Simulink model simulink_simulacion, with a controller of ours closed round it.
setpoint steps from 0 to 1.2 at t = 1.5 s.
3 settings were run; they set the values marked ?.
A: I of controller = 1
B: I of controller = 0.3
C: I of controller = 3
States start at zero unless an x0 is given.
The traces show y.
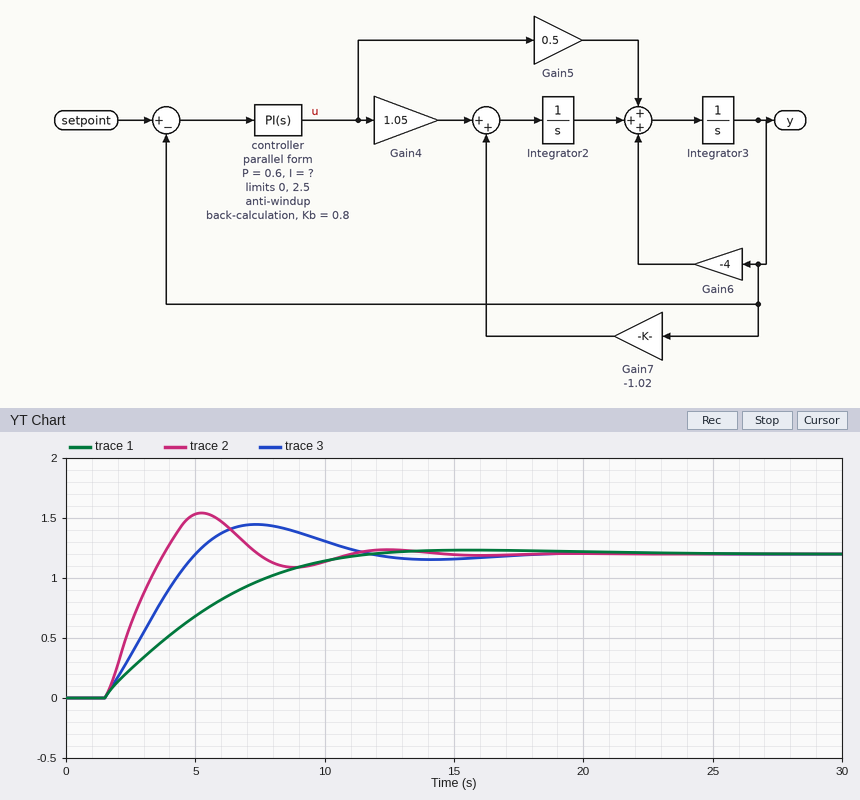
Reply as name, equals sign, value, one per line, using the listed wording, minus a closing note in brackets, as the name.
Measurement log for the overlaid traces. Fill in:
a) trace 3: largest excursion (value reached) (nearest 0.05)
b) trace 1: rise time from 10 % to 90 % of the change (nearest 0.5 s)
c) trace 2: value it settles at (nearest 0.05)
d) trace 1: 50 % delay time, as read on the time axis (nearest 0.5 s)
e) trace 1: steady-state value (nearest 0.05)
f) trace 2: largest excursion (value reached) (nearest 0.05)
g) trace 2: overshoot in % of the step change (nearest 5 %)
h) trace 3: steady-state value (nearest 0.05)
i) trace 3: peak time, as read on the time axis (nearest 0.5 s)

trace 3: largest excursion (value reached) = 1.45
trace 1: rise time from 10 % to 90 % of the change = 7.0 s
trace 2: value it settles at = 1.20
trace 1: 50 % delay time, as read on the time axis = 4.5 s
trace 1: steady-state value = 1.20
trace 2: largest excursion (value reached) = 1.55
trace 2: overshoot in % of the step change = 30 %
trace 3: steady-state value = 1.20
trace 3: peak time, as read on the time axis = 7.5 s
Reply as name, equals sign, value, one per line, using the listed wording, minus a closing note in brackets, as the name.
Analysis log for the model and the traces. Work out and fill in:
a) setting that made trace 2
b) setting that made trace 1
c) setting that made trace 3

setting that made trace 2 = C
setting that made trace 1 = B
setting that made trace 3 = A
